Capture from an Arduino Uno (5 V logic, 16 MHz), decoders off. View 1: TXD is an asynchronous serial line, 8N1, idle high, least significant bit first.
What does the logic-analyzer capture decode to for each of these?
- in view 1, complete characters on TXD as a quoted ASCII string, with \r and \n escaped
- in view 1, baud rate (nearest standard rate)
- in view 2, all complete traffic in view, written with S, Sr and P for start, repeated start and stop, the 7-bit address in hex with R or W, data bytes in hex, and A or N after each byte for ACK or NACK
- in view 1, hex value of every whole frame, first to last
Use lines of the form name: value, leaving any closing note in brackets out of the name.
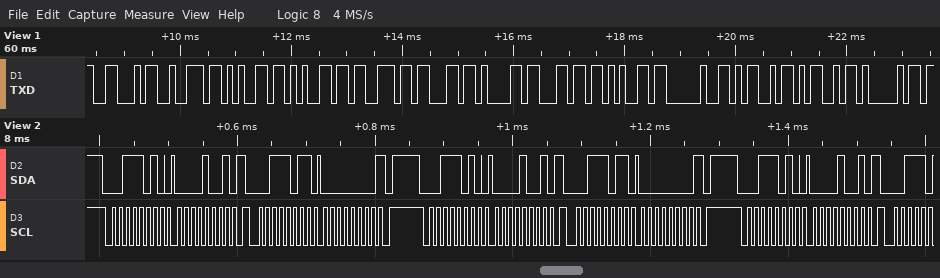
in view 1, complete characters on TXD as a quoted ASCII string, with \r and \n escaped: "Freescale MMA"
in view 1, baud rate: 9600 baud
in view 2, all complete traffic in view, written with S, Sr and P for start, repeated start and stop, the 7-bit address in hex with R or W, data bytes in hex, and A or N after each byte for ACK or NACK: S 1DW A 09 A Sr 1DR A 00 N P S 1DW A 09 A Sr 1DR A 00 N P S 1DW A 09 A
in view 1, hex value of every whole frame, first to last: 46 72 65 65 73 63 61 6C 65 20 4D 4D 41
